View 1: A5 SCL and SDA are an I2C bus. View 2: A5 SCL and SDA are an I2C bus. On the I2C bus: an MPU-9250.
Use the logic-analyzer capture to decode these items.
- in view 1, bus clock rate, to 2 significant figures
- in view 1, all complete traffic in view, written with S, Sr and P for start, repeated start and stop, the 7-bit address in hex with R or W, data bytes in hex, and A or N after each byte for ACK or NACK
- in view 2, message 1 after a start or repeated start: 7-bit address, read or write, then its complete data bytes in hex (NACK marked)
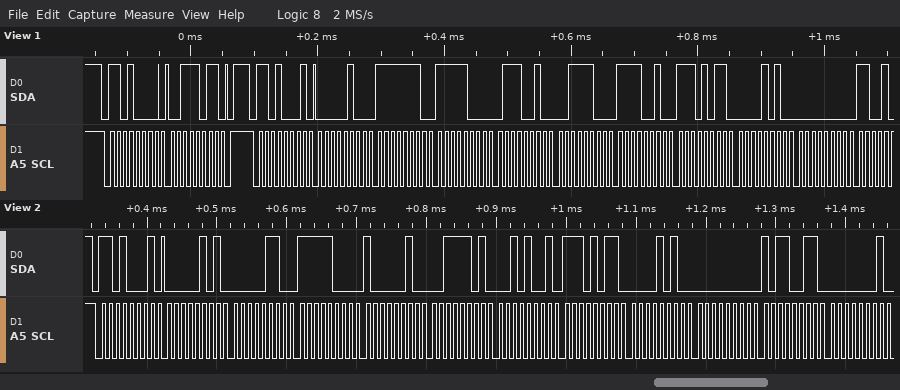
100 kHz
S 68W A 3B A P S 68R A 04 A FE A F8 A 72 A 3C A F2 A EB A 0A A 00 A
0x68 read: 05 06 F8 82 3D 29 EB 0A 00 B3 01
